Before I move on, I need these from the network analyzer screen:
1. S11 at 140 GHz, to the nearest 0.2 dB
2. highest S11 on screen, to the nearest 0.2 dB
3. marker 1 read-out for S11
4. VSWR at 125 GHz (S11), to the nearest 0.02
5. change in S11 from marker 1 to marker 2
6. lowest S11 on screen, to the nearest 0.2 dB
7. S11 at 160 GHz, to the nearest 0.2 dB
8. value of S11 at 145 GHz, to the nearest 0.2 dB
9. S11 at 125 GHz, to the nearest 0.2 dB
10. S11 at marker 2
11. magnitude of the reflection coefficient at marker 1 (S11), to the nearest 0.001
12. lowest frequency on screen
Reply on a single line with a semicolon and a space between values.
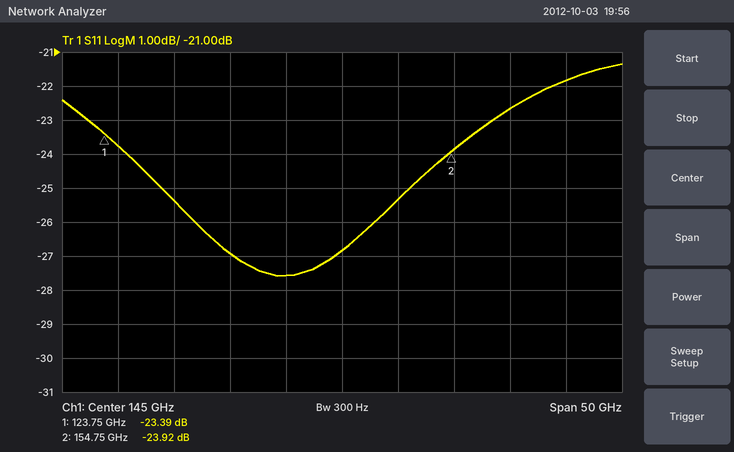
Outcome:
-27.6 dB; -21.4 dB; -23.39 dB; 1.14; -0.53 dB; -27.6 dB; -22.6 dB; -26.8 dB; -23.8 dB; -23.92 dB; 0.068; 120 GHz
